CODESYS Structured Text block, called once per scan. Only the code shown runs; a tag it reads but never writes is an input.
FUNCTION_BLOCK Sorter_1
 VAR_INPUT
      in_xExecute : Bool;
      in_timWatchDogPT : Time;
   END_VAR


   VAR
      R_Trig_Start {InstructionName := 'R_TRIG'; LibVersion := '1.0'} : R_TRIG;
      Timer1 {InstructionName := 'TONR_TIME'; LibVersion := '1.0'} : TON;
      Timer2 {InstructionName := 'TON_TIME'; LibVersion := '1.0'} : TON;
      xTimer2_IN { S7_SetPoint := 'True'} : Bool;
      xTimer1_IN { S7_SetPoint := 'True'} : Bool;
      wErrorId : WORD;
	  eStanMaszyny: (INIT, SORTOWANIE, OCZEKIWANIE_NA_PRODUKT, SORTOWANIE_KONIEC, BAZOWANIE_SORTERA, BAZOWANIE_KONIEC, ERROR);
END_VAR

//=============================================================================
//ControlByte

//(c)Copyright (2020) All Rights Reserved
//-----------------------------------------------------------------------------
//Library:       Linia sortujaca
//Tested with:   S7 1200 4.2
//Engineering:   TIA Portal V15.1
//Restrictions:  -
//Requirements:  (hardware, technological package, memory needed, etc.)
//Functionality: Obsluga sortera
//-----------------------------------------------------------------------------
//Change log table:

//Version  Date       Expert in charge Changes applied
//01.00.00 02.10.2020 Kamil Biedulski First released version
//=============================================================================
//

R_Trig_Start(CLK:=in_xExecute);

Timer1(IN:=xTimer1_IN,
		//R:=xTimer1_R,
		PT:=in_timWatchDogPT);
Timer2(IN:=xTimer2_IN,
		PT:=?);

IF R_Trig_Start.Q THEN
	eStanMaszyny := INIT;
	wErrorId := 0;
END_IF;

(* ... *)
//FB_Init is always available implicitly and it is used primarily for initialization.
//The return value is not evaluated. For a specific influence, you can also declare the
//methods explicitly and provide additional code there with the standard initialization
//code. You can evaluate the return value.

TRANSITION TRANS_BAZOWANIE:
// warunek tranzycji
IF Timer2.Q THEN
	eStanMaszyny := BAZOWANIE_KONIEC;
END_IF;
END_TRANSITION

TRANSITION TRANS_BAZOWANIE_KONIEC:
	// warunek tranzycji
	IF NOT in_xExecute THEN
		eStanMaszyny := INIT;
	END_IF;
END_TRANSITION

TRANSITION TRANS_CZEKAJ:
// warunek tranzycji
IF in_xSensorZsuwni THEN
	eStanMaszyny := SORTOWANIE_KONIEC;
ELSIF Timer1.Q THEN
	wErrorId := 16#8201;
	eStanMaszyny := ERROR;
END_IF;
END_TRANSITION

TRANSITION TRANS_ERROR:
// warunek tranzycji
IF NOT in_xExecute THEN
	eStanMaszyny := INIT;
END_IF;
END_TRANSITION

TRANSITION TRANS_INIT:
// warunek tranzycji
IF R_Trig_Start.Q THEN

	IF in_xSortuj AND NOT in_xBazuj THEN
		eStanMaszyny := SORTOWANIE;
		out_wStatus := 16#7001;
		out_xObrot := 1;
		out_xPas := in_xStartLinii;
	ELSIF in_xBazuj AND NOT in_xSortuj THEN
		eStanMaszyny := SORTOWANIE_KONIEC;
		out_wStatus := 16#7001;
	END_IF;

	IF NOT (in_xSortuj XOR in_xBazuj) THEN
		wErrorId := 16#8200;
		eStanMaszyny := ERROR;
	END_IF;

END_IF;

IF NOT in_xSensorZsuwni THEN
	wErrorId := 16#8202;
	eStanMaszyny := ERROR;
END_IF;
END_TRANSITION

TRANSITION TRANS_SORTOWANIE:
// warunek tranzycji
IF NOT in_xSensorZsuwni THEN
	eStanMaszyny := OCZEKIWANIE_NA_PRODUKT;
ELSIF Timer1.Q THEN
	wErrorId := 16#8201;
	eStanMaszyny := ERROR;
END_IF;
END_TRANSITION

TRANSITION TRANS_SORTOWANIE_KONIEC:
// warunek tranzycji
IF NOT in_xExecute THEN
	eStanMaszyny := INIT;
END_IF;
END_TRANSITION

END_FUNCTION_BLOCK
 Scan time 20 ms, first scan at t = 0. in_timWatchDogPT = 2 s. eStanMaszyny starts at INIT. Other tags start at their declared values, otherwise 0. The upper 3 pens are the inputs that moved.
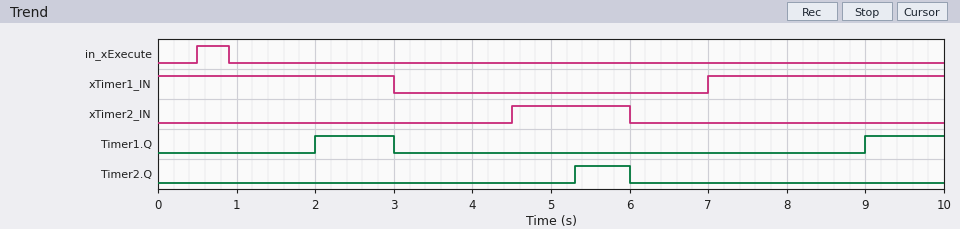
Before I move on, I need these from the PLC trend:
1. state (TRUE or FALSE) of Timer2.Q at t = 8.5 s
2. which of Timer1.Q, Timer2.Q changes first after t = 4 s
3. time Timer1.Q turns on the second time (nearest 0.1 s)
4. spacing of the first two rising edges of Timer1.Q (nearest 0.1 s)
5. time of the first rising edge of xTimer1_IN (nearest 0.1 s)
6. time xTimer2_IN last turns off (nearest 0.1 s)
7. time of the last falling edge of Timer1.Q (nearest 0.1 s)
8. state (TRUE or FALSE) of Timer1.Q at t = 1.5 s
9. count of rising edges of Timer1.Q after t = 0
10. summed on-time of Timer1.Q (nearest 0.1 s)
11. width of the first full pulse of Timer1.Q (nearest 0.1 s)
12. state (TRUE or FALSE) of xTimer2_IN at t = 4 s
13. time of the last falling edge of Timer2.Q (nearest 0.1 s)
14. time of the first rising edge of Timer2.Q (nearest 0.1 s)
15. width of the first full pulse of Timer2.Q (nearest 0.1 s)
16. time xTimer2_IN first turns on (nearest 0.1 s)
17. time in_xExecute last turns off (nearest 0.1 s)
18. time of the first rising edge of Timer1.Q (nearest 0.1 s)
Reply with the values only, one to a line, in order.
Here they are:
FALSE
Timer2.Q
9.0 s
7.0 s
7.0 s
6.0 s
3.0 s
FALSE
2
2.0 s
1.0 s
FALSE
6.0 s
5.3 s
0.7 s
4.5 s
0.9 s
2.0 s
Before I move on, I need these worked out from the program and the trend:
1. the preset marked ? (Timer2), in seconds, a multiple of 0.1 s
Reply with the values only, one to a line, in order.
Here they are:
0.8 s
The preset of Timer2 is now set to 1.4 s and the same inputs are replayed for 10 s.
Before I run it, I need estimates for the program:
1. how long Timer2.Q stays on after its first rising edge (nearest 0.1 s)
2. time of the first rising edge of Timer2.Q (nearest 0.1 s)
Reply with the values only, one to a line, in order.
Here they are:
0.1 s
5.9 s
